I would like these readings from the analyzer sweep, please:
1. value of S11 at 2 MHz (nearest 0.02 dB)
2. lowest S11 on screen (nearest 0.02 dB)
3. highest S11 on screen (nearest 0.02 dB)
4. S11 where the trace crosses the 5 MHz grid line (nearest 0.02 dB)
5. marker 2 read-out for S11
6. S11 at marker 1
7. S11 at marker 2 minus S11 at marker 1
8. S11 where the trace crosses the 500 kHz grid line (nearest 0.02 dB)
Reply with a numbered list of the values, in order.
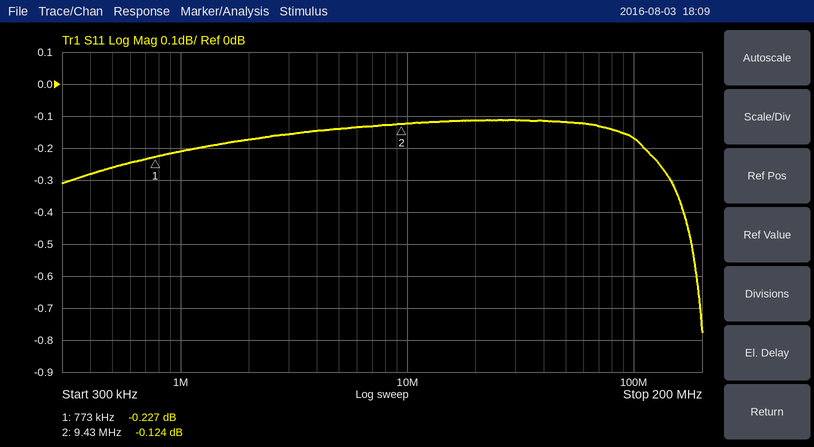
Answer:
1. -0.18 dB
2. -0.78 dB
3. -0.12 dB
4. -0.14 dB
5. -0.124 dB
6. -0.227 dB
7. 0.103 dB
8. -0.26 dB
